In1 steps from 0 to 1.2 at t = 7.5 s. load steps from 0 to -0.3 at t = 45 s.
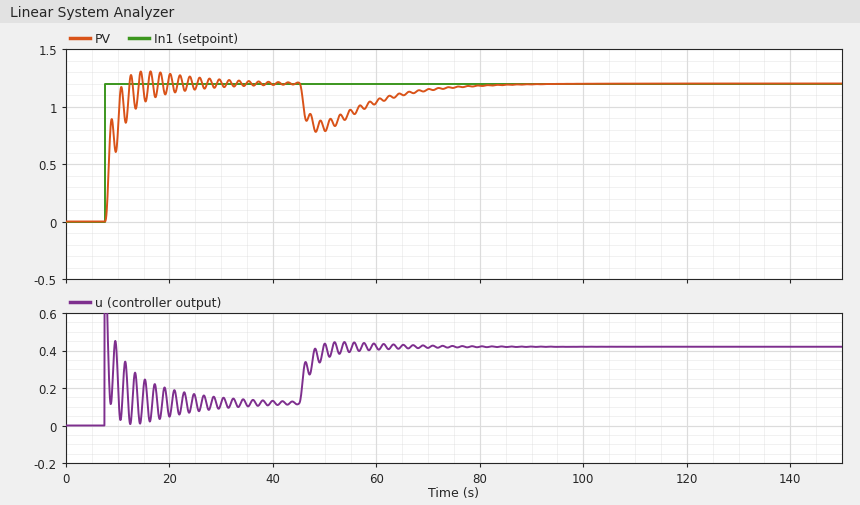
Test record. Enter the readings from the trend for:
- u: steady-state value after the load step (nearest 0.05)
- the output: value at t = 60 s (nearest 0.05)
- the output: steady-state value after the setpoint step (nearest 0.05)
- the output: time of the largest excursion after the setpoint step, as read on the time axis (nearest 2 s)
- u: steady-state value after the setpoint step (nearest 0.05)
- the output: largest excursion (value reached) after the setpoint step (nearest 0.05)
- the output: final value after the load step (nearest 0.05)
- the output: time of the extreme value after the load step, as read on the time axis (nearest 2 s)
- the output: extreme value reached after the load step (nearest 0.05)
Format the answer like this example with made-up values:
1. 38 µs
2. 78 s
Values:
1. 0.40
2. 1.05
3. 1.20
4. 16 s
5. 0.10
6. 1.30
7. 1.20
8. 48 s
9. 0.80
